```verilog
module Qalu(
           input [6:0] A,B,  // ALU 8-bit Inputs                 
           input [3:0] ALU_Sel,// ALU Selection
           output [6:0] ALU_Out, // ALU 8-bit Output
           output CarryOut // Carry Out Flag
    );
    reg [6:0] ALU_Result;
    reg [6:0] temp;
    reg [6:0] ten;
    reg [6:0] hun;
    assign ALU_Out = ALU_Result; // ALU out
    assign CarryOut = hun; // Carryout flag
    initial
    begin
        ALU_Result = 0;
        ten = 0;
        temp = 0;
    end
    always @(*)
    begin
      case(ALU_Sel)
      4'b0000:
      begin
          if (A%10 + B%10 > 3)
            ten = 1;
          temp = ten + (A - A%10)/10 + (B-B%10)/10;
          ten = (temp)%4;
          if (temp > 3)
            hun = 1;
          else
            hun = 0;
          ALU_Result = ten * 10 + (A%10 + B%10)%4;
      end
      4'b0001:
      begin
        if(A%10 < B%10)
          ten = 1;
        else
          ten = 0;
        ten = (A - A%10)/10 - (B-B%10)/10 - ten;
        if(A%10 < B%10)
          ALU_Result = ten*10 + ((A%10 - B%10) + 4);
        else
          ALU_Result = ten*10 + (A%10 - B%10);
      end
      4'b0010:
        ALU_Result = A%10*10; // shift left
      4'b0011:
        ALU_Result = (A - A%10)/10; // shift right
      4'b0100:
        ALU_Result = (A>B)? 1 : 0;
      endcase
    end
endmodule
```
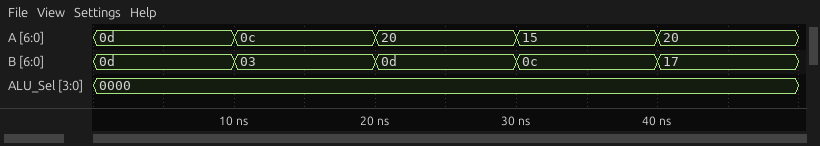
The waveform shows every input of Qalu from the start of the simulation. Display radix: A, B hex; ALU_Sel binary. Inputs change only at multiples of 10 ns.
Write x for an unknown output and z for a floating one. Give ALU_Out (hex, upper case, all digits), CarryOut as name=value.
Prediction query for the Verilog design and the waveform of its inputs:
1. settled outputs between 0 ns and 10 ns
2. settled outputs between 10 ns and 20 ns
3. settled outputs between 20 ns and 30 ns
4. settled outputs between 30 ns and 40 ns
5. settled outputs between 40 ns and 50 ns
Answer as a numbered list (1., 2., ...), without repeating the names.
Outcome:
1. ALU_Out=20, CarryOut=0
2. ALU_Out=15, CarryOut=0
3. ALU_Out=0B, CarryOut=1
4. ALU_Out=03, CarryOut=1
5. ALU_Out=15, CarryOut=1
